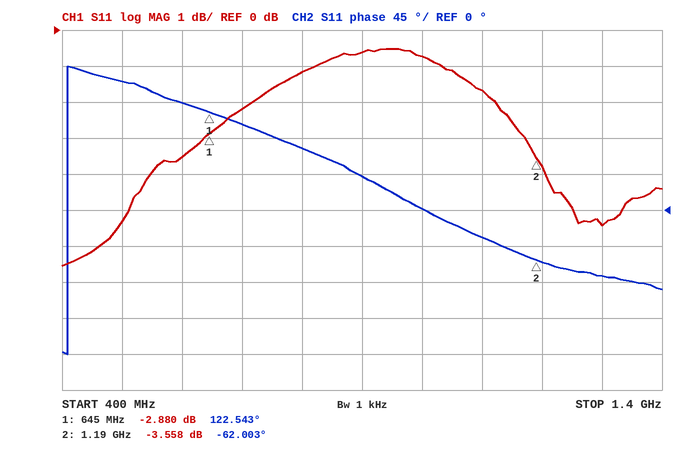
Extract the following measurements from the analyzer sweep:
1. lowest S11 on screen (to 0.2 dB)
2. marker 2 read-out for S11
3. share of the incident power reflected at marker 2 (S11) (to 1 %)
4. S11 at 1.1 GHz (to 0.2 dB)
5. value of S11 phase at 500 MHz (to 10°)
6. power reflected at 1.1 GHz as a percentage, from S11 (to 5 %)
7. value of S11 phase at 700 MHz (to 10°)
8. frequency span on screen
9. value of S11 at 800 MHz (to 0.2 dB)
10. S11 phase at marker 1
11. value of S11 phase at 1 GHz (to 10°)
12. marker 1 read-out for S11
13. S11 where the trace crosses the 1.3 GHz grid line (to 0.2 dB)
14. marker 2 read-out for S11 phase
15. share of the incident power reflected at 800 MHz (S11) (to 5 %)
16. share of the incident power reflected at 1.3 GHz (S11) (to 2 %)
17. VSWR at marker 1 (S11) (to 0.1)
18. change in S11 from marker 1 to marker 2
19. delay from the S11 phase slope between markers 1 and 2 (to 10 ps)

-6.6 dB
-3.558 dB
44 %
-1.6 dB
160°
70 %
110°
1 GHz
-1.2 dB
122.543°
0°
-2.880 dB
-5.4 dB
-62.003°
75 %
28 %
6.1
-0.678 dB
940 ps
